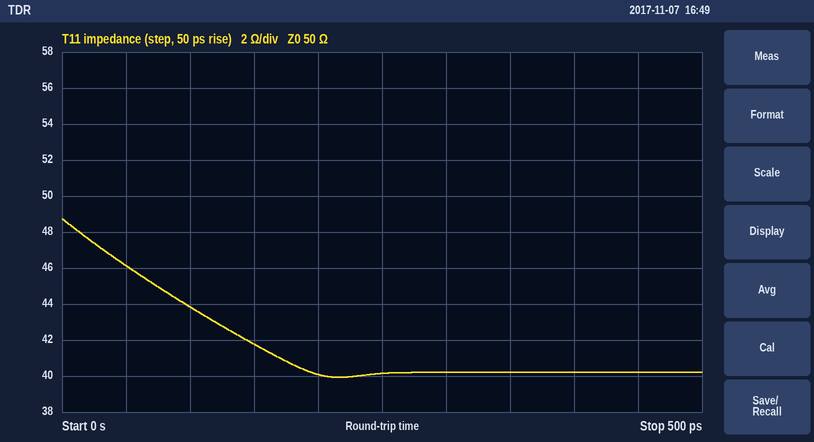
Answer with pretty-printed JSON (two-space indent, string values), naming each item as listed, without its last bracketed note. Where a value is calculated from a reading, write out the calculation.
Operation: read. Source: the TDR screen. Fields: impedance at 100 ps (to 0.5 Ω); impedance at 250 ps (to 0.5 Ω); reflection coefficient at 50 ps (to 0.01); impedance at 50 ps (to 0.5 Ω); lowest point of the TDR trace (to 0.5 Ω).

{
  "impedance at 100 ps": "44.0 Ω",
  "impedance at 250 ps": "40.0 Ω",
  "reflection coefficient at 50 ps": "(46 − 50)/(46 + 50) ≈ -0.04",
  "impedance at 50 ps": "46.0 Ω",
  "lowest point of the TDR trace": "40.0 Ω"
}
